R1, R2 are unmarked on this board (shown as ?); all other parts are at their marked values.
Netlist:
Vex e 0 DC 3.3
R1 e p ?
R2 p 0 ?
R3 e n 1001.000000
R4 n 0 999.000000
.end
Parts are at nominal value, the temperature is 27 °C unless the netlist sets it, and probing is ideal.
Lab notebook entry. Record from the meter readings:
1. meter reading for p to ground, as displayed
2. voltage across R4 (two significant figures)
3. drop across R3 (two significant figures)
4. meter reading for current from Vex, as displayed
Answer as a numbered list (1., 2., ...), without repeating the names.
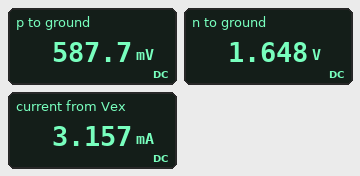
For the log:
1. 587.7 mV
2. 1.6 V
3. 1.7 V
4. 3.157 mA
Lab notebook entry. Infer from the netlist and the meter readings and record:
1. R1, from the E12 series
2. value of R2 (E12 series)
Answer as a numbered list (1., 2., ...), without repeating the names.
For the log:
1. 1.8 kΩ
2. 390 Ω
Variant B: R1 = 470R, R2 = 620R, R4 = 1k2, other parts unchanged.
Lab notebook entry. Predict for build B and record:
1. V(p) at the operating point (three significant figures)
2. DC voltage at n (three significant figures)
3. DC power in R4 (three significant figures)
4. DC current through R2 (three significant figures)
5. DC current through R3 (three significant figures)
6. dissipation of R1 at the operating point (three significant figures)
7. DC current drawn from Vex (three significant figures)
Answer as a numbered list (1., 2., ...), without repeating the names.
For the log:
1. 1.88 V
2. 1.80 V
3. 2.70 mW
4. 3.03 mA
5. 1.50 mA
6. 4.31 mW
7. 4.53 mA
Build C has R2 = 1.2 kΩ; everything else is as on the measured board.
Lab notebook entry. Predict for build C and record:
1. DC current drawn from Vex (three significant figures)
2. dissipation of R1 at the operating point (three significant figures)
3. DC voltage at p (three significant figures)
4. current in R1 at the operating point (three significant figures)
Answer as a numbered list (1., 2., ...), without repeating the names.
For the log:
1. 2.75 mA
2. 2.18 mW
3. 1.32 V
4. 1.10 mA
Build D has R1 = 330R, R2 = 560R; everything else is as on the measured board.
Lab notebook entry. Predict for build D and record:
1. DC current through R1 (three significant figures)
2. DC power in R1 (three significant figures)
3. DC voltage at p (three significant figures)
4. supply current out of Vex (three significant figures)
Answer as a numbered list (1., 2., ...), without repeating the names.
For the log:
1. 3.71 mA
2. 4.54 mW
3. 2.08 V
4. 5.36 mA
